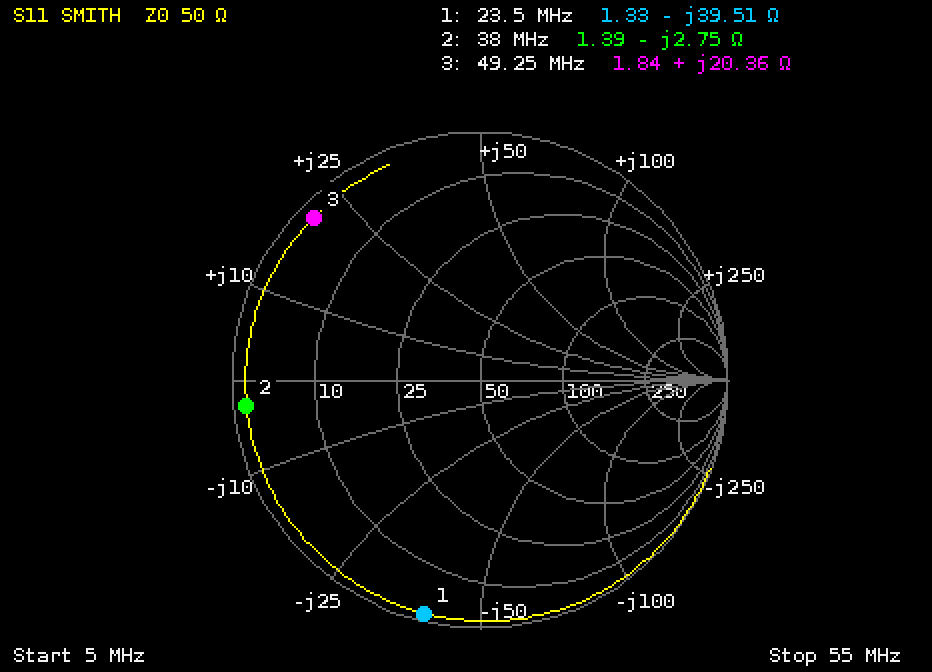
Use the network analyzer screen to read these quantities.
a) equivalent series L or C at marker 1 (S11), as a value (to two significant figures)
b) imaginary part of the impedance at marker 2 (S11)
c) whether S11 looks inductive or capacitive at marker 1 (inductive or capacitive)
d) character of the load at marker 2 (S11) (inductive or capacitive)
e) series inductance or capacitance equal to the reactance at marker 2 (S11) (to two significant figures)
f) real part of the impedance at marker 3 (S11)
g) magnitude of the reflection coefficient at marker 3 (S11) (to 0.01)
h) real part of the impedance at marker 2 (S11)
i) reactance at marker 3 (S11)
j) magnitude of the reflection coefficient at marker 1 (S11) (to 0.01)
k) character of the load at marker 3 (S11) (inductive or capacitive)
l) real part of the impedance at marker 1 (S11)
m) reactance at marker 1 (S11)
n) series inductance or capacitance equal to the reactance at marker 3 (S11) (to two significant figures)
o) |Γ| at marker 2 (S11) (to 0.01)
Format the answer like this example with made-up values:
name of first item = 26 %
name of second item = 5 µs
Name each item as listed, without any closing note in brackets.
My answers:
equivalent series L or C at marker 1 (S11), as a value = 170 pF
imaginary part of the impedance at marker 2 = -2.75 Ω
whether S11 looks inductive or capacitive at marker 1 = capacitive
character of the load at marker 2 (S11) = capacitive
series inductance or capacitance equal to the reactance at marker 2 (S11) = 1.5 nF
real part of the impedance at marker 3 = 1.84 Ω
magnitude of the reflection coefficient at marker 3 (S11) = 0.94
real part of the impedance at marker 2 = 1.39 Ω
reactance at marker 3 = +20.36 Ω
magnitude of the reflection coefficient at marker 1 (S11) = 0.97
character of the load at marker 3 (S11) = inductive
real part of the impedance at marker 1 = 1.33 Ω
reactance at marker 1 = -39.51 Ω
series inductance or capacitance equal to the reactance at marker 3 (S11) = 66 nH
|Γ| at marker 2 (S11) = 0.95
